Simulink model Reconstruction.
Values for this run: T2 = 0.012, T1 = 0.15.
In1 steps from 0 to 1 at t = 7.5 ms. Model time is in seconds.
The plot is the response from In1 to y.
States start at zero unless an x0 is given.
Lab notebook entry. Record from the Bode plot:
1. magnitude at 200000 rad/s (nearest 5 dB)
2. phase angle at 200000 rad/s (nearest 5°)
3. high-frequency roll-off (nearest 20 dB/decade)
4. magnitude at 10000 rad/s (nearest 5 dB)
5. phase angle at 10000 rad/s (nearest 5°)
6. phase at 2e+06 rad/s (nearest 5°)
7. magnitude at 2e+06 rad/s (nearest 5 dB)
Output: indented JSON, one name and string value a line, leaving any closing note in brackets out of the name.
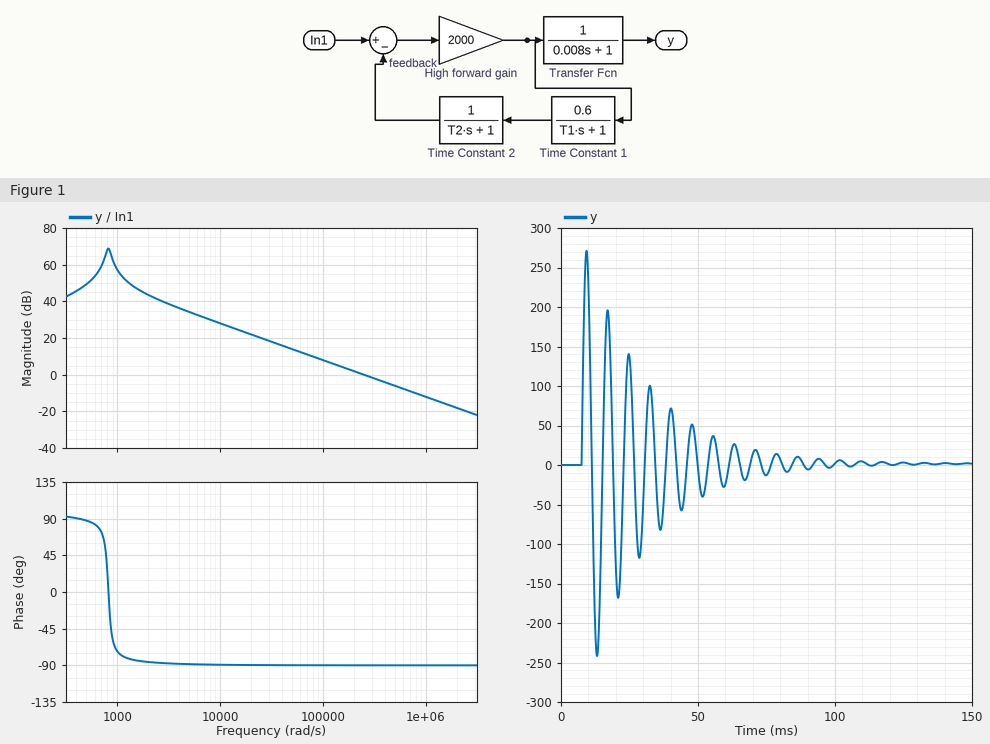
{
  "magnitude at 200000 rad/s": "0 dB",
  "phase angle at 200000 rad/s": "-90°",
  "high-frequency roll-off": "-20 dB/decade",
  "magnitude at 10000 rad/s": "30 dB",
  "phase angle at 10000 rad/s": "-90°",
  "phase at 2e+06 rad/s": "-90°",
  "magnitude at 2e+06 rad/s": "-20 dB"
}
